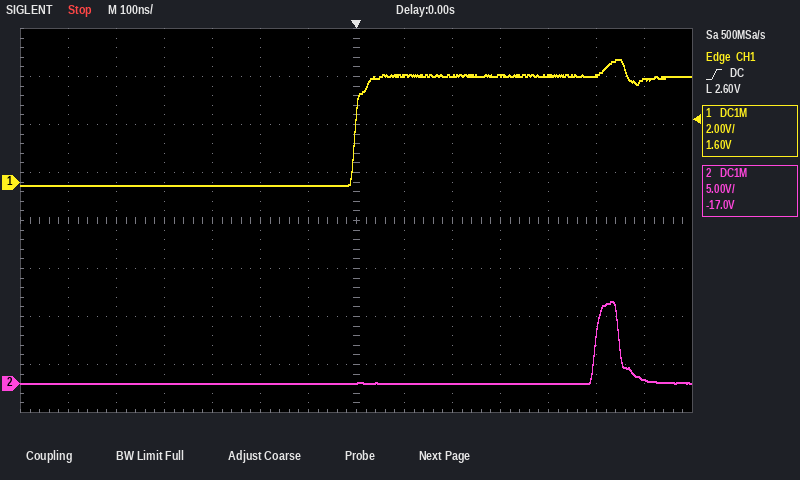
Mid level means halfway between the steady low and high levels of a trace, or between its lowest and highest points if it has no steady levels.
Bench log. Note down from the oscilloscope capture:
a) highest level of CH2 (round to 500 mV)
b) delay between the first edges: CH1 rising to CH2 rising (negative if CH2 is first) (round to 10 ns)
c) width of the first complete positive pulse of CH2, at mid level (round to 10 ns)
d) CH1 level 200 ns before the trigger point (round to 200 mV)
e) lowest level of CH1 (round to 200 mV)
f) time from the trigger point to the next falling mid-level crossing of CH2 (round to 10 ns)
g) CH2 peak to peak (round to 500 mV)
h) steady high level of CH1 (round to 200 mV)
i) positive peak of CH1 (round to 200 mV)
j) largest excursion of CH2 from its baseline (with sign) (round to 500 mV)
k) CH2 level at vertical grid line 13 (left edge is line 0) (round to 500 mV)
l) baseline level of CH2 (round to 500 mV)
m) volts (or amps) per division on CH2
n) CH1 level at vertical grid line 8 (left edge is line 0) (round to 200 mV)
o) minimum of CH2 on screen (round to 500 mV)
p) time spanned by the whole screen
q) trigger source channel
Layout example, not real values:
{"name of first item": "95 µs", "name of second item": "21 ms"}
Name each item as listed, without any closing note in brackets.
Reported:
{"highest level of CH2": "8.5 V", "delay between the first edges: CH1 rising to CH2 rising (negative if CH2 is first)": "+500 ns", "width of the first complete positive pulse of CH2, at mid level": "50 ns", "CH1 level 200 ns before the trigger point": "-200 mV", "lowest level of CH1": "-200 mV", "time from the trigger point to the next falling mid-level crossing of CH2": "550 ns", "CH2 peak to peak": "8.5 V", "steady high level of CH1": "4.4 V", "positive peak of CH1": "5.2 V", "largest excursion of CH2 from its baseline (with sign)": "+8.5 V", "CH2 level at vertical grid line 13 (left edge is line 0)": "500 mV", "baseline level of CH2": "0.0 V", "volts (or amps) per division on CH2": "5 V", "CH1 level at vertical grid line 8 (left edge is line 0)": "4.4 V", "minimum of CH2 on screen": "0.0 V", "time spanned by the whole screen": "1.4 µs", "trigger source channel": "CH1"}
